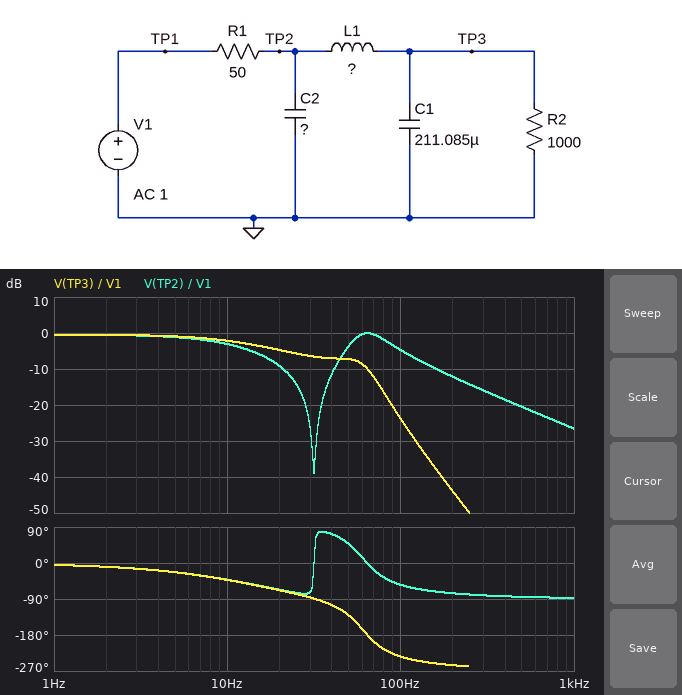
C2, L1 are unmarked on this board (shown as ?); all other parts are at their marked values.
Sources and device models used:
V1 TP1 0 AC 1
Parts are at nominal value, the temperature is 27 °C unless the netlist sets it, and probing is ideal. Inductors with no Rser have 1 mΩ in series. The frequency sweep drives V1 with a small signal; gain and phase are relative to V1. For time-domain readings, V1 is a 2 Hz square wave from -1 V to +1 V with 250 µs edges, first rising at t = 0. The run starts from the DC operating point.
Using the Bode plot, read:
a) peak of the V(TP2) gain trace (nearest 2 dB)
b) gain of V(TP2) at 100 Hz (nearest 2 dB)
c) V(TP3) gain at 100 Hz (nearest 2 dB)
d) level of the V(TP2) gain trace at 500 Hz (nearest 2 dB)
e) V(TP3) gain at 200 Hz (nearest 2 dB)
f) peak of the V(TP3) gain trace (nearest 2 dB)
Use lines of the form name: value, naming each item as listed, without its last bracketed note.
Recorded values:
peak of the V(TP2) gain trace: 0 dB
gain of V(TP2) at 100 Hz: -4 dB
V(TP3) gain at 100 Hz: -24 dB
level of the V(TP2) gain trace at 500 Hz: -20 dB
V(TP3) gain at 200 Hz: -44 dB
peak of the V(TP3) gain trace: 0 dB
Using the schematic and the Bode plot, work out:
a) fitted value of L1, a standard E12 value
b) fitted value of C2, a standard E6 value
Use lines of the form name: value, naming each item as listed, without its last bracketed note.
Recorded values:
fitted value of L1, a standard E12 value: 120 mH
fitted value of C2, a standard E6 value: 68 µF
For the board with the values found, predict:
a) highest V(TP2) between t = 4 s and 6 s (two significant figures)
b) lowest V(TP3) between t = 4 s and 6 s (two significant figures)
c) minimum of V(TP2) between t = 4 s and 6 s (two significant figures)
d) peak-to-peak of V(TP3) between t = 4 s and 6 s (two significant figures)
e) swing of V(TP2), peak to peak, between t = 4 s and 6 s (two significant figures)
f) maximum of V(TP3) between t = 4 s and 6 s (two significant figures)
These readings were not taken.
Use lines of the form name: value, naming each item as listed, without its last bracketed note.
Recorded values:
highest V(TP2) between t = 4 s and 6 s: 950 mV
lowest V(TP3) between t = 4 s and 6 s: -950 mV
minimum of V(TP2) between t = 4 s and 6 s: -950 mV
peak-to-peak of V(TP3) between t = 4 s and 6 s: 1.9 V
swing of V(TP2), peak to peak, between t = 4 s and 6 s: 1.9 V
maximum of V(TP3) between t = 4 s and 6 s: 950 mV
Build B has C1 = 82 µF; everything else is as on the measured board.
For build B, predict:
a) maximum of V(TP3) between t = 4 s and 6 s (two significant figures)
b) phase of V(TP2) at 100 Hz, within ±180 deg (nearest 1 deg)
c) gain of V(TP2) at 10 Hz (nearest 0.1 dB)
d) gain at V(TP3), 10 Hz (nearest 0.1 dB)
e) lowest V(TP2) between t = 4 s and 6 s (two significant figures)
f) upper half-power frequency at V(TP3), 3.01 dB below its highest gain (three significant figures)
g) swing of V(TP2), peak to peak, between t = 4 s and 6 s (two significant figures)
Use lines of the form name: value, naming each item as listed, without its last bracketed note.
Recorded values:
maximum of V(TP3) between t = 4 s and 6 s: 1.0 V
phase of V(TP2) at 100 Hz, within ±180 deg: -51 deg
gain of V(TP2) at 10 Hz: -1.3 dB
gain at V(TP3), 10 Hz: -0.9 dB
lowest V(TP2) between t = 4 s and 6 s: -1.0 V
upper half-power frequency at V(TP3), 3.01 dB below its highest gain: 78.6 Hz
swing of V(TP2), peak to peak, between t = 4 s and 6 s: 2.0 V
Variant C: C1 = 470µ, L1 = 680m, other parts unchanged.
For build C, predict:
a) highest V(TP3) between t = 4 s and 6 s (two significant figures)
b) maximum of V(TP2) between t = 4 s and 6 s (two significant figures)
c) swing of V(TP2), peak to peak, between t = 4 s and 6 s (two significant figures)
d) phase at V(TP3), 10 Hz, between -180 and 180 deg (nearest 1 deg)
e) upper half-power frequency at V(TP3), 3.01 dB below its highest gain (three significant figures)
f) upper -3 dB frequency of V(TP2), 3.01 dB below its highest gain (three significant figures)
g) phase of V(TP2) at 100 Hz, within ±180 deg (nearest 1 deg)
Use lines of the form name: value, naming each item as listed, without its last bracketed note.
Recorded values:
highest V(TP3) between t = 4 s and 6 s: 1.0 V
maximum of V(TP2) between t = 4 s and 6 s: 990 mV
swing of V(TP2), peak to peak, between t = 4 s and 6 s: 2.0 V
phase at V(TP3), 10 Hz, between -180 and 180 deg: -99 deg
upper half-power frequency at V(TP3), 3.01 dB below its highest gain: 10.0 Hz
upper -3 dB frequency of V(TP2), 3.01 dB below its highest gain: 56.8 Hz
phase of V(TP2) at 100 Hz, within ±180 deg: -64 deg
